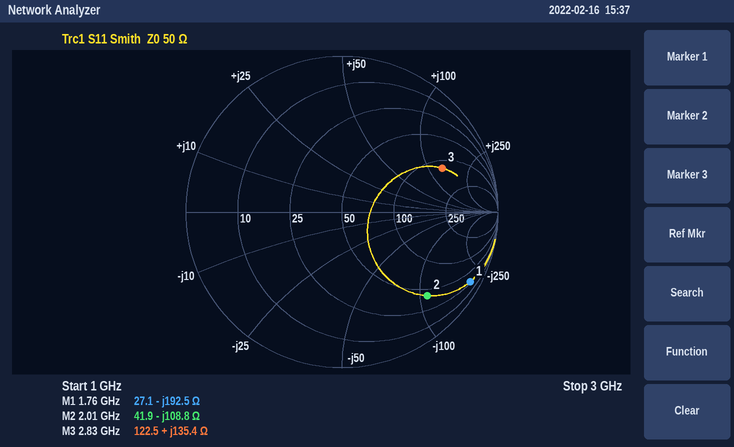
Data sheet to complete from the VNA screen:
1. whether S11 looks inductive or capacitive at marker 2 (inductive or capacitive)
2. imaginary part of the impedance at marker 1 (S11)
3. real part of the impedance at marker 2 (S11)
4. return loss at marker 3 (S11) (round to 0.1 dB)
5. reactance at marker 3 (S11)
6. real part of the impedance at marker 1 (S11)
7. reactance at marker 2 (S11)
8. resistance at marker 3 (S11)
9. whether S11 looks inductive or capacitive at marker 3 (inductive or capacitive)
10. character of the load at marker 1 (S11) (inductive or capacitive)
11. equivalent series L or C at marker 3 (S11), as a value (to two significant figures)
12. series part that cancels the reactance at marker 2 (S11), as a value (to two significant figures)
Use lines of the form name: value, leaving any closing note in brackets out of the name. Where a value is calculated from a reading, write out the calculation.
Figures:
whether S11 looks inductive or capacitive at marker 2: capacitive
imaginary part of the impedance at marker 1: -192.5 Ω
real part of the impedance at marker 2: 41.9 Ω
return loss at marker 3 (S11): 3.1 dB
reactance at marker 3: +135.4 Ω
real part of the impedance at marker 1: 27.1 Ω
reactance at marker 2: -108.8 Ω
resistance at marker 3: 122.5 Ω
whether S11 looks inductive or capacitive at marker 3: inductive
character of the load at marker 1 (S11): capacitive
equivalent series L or C at marker 3 (S11), as a value: L = 135.4 Ω/(2π × 2.83 GHz) ≈ 7.6 nH
series part that cancels the reactance at marker 2 (S11), as a value: L = 108.8 Ω/(2π × 2.01 GHz) ≈ 8.6 nH
